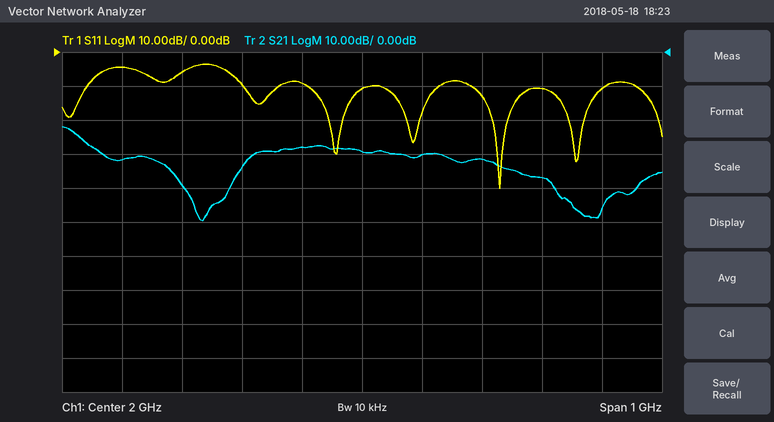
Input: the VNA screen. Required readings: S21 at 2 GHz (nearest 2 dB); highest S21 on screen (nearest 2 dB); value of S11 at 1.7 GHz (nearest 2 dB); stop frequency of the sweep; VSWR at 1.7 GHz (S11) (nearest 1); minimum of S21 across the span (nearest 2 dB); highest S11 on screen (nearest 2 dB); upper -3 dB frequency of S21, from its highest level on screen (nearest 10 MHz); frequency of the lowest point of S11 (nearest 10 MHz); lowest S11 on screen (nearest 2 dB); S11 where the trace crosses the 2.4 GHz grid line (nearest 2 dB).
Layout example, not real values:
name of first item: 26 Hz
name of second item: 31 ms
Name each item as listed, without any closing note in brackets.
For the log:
S21 at 2 GHz: -30 dB
highest S21 on screen: -22 dB
value of S11 at 1.7 GHz: -6 dB
stop frequency of the sweep: 2.5 GHz
VSWR at 1.7 GHz (S11): 3
minimum of S21 across the span: -50 dB
highest S11 on screen: -4 dB
upper -3 dB frequency of S21, from its highest level on screen: 1.53 GHz
frequency of the lowest point of S11: 2.23 GHz
lowest S11 on screen: -40 dB
S11 where the trace crosses the 2.4 GHz grid line: -10 dB
